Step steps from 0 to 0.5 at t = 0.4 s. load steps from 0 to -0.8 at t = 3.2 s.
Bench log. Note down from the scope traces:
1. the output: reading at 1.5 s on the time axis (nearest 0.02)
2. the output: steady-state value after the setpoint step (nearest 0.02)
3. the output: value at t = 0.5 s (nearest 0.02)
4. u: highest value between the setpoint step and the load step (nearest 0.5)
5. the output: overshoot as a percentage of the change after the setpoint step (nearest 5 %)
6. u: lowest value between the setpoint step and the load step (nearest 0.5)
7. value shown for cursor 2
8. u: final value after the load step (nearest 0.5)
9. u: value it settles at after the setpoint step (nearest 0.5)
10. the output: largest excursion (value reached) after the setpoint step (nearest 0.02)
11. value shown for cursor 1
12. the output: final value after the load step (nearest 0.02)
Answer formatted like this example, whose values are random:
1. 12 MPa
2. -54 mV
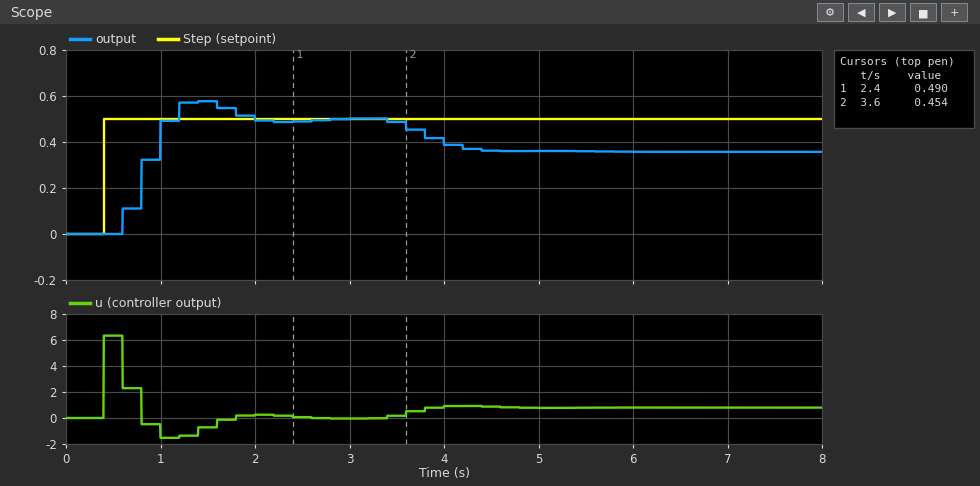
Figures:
1. 0.58
2. 0.50
3. 0.00
4. 6.5
5. 15 %
6. -1.5
7. 0.454
8. 1.0
9. 0.0
10. 0.58
11. 0.490
12. 0.36
